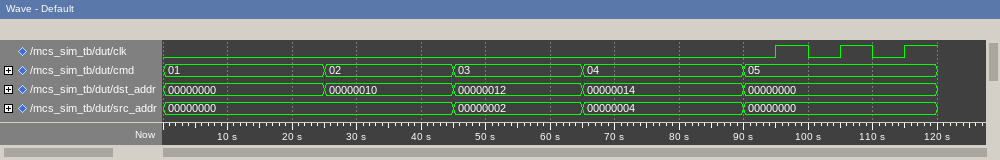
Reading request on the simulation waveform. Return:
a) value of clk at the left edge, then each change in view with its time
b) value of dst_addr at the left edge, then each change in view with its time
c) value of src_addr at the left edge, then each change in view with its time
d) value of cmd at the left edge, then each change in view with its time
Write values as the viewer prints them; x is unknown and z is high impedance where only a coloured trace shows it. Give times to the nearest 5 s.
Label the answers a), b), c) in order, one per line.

a) 0, 1 at 95 s, 0 at 100 s, 1 at 105 s, 0 at 110 s, 1 at 115 s
b) 00000000, 00000010 at 25 s, 00000012 at 45 s, 00000014 at 65 s, 00000000 at 90 s
c) 00000000, 00000002 at 45 s, 00000004 at 65 s, 00000000 at 90 s
d) 01, 02 at 25 s, 03 at 45 s, 04 at 65 s, 05 at 90 s
